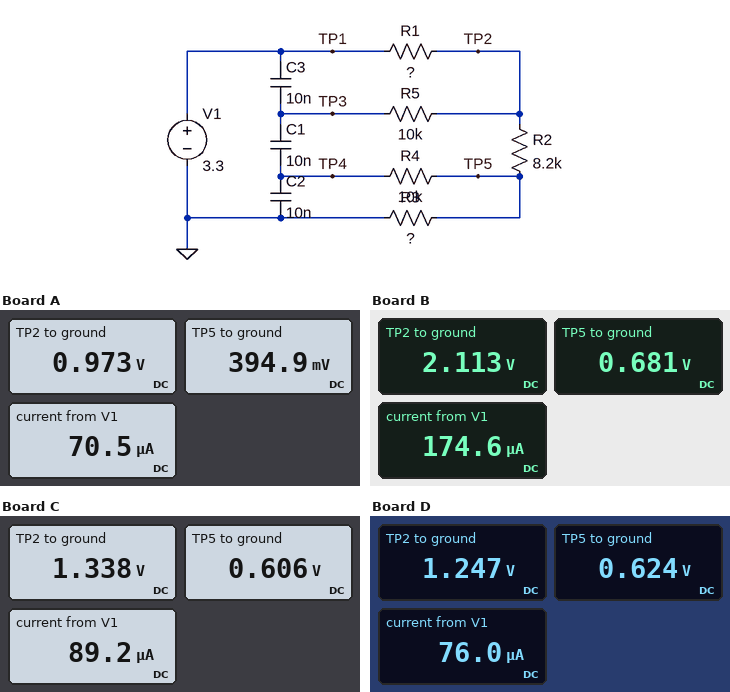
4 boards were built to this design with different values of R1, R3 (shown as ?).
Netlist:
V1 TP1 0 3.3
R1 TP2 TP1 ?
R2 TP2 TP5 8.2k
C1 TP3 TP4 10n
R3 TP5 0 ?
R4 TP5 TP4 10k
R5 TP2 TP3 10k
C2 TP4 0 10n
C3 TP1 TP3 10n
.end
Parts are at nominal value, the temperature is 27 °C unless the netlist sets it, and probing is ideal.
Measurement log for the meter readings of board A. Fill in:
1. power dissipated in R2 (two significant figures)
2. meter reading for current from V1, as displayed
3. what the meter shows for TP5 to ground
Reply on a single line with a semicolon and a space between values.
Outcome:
41 µW; 70.5 µA; 394.9 mV
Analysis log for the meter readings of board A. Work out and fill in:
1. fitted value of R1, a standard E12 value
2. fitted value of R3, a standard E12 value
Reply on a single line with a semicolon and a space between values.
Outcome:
33 kΩ; 5.6 kΩ
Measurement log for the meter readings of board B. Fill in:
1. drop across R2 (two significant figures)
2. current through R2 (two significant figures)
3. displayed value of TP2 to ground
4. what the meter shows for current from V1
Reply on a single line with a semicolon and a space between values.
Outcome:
1.4 V; 170 µA; 2.113 V; 174.6 µA
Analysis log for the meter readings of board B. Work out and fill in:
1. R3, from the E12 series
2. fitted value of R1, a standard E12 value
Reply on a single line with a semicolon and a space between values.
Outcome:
3.9 kΩ; 6.8 kΩ
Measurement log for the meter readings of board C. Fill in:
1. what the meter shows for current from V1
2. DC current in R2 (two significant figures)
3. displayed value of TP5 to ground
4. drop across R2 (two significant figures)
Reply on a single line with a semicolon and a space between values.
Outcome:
89.2 µA; 89 µA; 0.606 V; 730 mV
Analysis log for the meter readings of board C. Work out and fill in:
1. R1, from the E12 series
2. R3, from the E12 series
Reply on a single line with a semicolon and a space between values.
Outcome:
22 kΩ; 6.8 kΩ
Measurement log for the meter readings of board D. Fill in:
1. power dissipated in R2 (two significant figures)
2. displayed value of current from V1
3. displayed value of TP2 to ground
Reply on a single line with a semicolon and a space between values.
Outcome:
47 µW; 76.0 µA; 1.247 V
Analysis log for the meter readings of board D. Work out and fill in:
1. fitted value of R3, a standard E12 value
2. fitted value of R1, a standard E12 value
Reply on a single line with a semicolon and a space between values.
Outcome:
8.2 kΩ; 27 kΩ
